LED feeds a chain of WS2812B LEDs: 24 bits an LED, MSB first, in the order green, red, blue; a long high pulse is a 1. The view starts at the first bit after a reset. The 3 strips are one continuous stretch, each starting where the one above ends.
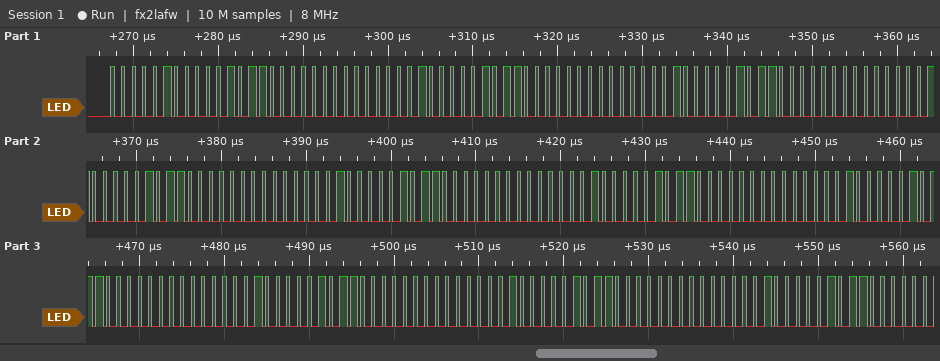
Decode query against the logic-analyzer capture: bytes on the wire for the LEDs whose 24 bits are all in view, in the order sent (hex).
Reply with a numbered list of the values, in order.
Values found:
1. 04 16 00 04 16 00 04 16 00 04 16 00 04 16 00 04 16 00 04 16 00 04 16 00 04 16 00
